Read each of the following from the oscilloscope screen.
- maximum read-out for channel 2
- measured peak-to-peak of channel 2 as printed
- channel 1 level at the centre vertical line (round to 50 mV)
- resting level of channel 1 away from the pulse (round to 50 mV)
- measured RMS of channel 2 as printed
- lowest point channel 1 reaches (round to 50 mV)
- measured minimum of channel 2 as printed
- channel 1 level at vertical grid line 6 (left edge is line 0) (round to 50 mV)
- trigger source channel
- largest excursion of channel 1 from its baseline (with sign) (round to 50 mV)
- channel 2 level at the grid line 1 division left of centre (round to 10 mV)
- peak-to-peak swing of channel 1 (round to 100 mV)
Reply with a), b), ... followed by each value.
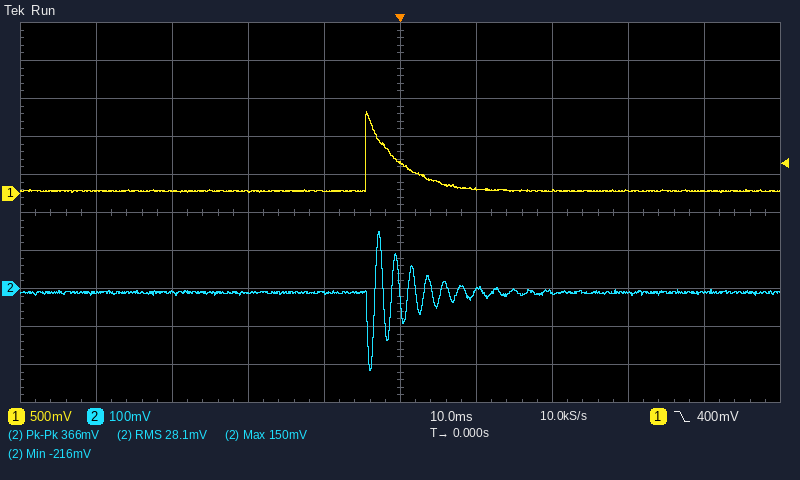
a) 150 mV
b) 366 mV
c) 400 mV
d) 50 mV
e) 28.1 mV
f) 0 mV
g) -216 mV
h) 50 mV
i) channel 1
j) +1.05 V
k) -10 mV
l) 1.10 V
